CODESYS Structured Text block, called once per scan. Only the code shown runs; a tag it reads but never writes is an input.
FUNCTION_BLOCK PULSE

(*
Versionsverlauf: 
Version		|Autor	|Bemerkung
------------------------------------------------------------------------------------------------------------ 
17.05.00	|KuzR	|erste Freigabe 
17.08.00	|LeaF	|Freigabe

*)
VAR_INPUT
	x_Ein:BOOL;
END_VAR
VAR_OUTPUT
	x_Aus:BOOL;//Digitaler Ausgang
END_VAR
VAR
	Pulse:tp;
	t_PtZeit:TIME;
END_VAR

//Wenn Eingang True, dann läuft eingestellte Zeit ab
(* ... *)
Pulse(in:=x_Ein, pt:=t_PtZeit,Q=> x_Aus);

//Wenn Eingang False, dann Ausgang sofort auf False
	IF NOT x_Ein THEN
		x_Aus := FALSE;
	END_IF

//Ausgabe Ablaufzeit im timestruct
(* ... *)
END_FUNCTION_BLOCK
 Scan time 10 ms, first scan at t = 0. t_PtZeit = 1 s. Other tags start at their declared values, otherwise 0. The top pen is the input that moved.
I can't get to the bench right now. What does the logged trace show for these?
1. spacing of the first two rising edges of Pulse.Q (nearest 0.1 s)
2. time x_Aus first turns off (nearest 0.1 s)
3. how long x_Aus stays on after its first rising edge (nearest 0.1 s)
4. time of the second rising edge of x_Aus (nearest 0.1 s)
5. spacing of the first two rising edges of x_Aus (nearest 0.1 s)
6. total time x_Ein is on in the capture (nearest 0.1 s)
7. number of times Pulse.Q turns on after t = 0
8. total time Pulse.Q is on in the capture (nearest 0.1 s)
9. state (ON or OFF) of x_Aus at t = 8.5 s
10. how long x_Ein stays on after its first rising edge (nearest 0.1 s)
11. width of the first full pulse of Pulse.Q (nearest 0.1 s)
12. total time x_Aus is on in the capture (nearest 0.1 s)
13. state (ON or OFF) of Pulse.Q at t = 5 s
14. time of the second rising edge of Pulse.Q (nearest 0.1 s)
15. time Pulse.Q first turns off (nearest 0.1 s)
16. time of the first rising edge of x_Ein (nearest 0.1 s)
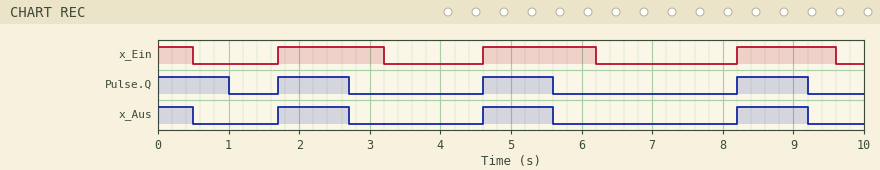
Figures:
2.9 s
0.5 s
1.0 s
4.6 s
2.9 s
5.0 s
3
4.0 s
ON
1.5 s
1.0 s
3.5 s
ON
4.6 s
1.0 s
1.7 s
